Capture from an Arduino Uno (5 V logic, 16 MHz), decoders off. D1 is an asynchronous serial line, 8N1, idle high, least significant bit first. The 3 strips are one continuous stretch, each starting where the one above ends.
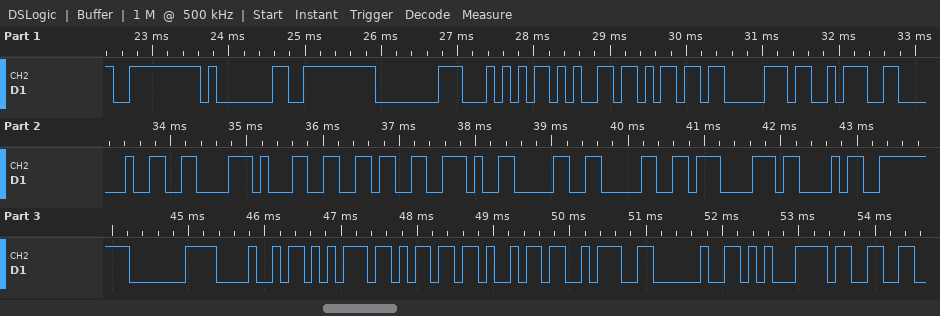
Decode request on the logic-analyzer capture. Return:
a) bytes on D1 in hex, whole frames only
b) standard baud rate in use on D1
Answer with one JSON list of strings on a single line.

["FE 01 FE 80 54 65 6D 70 3A 20 86 31 36 2E 30 30 87 43 FE C0 48 75 6D 69 3A 20 C5 33", "9600 baud"]
